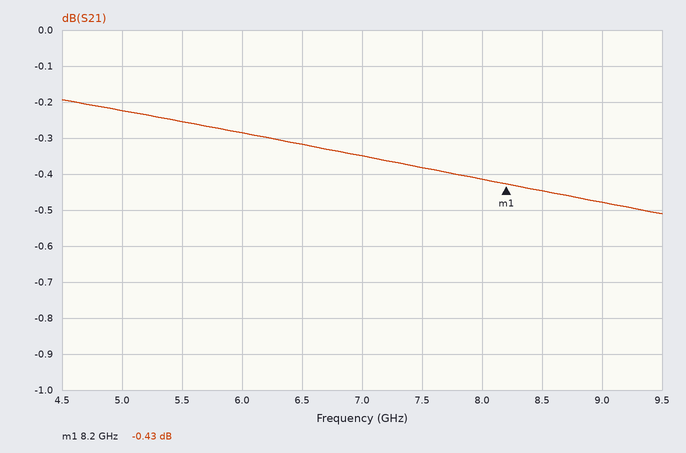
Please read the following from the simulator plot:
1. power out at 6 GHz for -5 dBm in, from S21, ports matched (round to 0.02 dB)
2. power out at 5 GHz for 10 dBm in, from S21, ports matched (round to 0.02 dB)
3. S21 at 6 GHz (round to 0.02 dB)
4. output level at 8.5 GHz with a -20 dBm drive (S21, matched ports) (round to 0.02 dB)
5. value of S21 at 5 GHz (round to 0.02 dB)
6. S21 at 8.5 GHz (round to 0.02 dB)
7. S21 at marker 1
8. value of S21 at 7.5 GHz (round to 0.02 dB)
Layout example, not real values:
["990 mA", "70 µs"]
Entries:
["-5.28 dBm", "9.78 dBm", "-0.28 dB", "-20.44 dBm", "-0.22 dB", "-0.44 dB", "-0.43 dB", "-0.38 dB"]
